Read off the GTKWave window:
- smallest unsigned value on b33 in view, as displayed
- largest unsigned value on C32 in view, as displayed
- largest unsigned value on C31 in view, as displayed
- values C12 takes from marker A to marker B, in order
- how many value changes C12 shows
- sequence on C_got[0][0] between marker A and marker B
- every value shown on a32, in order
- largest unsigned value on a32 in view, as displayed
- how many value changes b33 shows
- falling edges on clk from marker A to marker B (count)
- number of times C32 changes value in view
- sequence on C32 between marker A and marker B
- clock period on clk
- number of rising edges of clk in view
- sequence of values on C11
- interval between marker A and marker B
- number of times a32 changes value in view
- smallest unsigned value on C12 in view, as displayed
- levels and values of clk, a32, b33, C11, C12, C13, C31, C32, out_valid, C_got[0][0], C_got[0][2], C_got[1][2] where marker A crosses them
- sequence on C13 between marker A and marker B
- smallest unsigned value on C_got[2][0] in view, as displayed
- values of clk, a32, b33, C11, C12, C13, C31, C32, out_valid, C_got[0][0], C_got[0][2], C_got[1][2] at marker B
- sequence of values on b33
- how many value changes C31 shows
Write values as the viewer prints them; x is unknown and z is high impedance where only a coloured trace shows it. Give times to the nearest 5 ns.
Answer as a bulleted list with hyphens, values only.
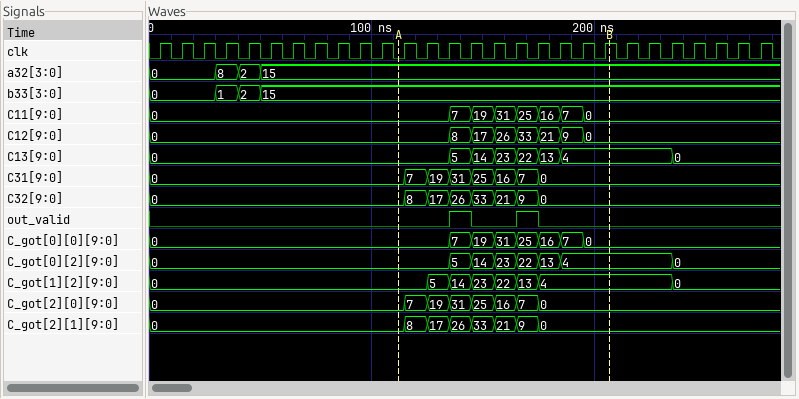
- 0
- 33
- 31
- 0, 8, 17, 26, 33, 21, 9, 0
- 7
- 0, 7, 19, 31, 25, 16, 7, 0
- 0, 8, 2, 15
- 15
- 3
- 9
- 7
- 0, 8, 17, 26, 33, 21, 9, 0
- 10 ns
- 28
- 0, 7, 19, 31, 25, 16, 7, 0
- 95 ns
- 3
- 0
- clk=0, a32=15, b33=15, C11=0, C12=0, C13=0, C31=0, C32=0, out_valid=0, C_got[0][0]=0, C_got[0][2]=0, C_got[1][2]=0
- 0, 5, 14, 23, 22, 13, 4
- 0
- clk=1, a32=15, b33=15, C11=0, C12=0, C13=4, C31=0, C32=0, out_valid=0, C_got[0][0]=0, C_got[0][2]=4, C_got[1][2]=4
- 0, 1, 2, 15
- 7
